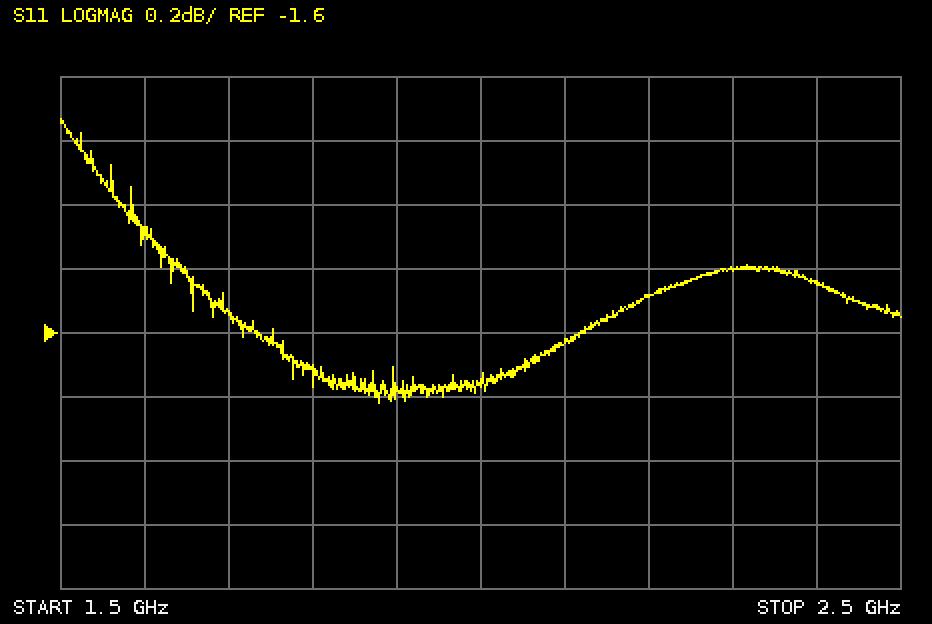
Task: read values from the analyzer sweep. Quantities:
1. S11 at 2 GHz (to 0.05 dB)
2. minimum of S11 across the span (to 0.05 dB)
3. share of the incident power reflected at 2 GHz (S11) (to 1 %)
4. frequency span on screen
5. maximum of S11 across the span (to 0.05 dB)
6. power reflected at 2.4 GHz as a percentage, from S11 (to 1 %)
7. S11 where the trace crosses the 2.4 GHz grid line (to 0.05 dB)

-1.75 dB
-1.80 dB
67 %
1 GHz
-0.95 dB
72 %
-1.45 dB
